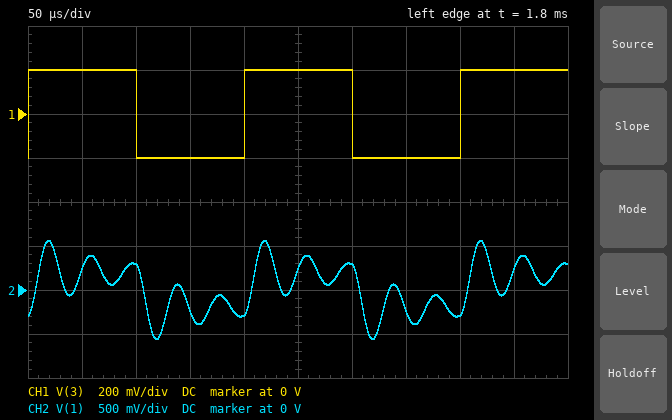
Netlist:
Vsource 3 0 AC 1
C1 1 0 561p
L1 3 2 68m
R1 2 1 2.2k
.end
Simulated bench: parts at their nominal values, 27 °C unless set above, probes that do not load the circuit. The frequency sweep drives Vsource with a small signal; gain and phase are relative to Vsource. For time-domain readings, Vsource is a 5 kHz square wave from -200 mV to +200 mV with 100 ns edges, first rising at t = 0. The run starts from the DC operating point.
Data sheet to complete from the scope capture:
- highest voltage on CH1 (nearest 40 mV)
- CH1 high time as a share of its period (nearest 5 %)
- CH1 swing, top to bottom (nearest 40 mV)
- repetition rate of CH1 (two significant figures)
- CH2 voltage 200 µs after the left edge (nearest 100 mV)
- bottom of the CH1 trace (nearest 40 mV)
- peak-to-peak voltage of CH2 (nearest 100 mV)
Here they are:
200 mV
50 %
400 mV
5.0 kHz
-300 mV
-200 mV
1.1 V
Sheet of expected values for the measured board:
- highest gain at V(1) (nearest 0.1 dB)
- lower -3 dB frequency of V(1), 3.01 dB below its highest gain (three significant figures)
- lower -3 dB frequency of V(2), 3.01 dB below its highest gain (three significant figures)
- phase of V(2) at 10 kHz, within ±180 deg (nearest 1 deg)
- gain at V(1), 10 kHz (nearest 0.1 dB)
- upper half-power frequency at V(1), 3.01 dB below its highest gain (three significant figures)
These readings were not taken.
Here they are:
14.0 dB
22.8 kHz
22.8 kHz
-1 deg
1.4 dB
28.0 kHz
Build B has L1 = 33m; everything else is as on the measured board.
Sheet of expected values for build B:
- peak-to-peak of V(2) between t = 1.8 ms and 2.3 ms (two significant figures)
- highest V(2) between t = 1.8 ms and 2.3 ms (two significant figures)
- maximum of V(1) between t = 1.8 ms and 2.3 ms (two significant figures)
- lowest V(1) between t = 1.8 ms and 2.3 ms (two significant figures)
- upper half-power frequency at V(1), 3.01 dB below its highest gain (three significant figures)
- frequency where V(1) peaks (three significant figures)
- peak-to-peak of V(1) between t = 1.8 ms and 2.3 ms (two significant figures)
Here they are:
940 mV
470 mV
460 mV
-460 mV
41.2 kHz
36.2 kHz
920 mV
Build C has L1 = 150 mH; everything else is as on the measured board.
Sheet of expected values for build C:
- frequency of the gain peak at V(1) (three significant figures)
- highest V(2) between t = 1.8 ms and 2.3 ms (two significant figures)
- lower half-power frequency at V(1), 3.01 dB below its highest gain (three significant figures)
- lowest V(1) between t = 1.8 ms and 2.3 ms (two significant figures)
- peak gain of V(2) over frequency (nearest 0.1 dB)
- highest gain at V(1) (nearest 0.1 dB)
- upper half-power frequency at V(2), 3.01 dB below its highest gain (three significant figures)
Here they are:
17.3 kHz
520 mV
16.1 kHz
-520 mV
17.5 dB
17.4 dB
18.4 kHz
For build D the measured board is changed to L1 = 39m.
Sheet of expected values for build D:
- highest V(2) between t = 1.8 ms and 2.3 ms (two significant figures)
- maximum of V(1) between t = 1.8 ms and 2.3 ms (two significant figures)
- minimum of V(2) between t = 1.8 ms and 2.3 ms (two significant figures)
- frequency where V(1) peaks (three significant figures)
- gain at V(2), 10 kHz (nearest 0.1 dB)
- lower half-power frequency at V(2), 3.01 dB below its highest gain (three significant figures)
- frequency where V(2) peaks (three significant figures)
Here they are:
480 mV
470 mV
-480 mV
33.4 kHz
0.8 dB
28.6 kHz
33.5 kHz
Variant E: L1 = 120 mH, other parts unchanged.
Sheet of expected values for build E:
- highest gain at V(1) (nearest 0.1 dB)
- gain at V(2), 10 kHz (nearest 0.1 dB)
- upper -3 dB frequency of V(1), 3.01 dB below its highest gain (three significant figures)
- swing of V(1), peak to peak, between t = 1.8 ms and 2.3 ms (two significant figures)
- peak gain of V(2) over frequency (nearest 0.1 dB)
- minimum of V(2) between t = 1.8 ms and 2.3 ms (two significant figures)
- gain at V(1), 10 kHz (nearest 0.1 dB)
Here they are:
16.5 dB
2.7 dB
20.7 kHz
860 mV
16.6 dB
-430 mV
2.6 dB
